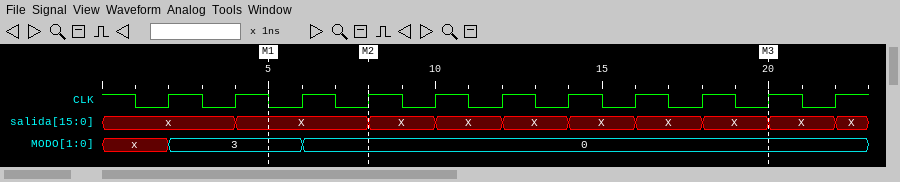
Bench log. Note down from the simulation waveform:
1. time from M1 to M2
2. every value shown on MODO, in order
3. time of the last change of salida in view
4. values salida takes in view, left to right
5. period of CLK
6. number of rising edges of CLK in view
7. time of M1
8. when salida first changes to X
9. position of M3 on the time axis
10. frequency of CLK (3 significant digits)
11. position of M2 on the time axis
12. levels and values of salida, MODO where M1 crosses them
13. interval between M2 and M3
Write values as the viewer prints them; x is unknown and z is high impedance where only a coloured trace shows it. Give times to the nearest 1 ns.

3 ns
x, 3, 0
22 ns
x, X, X, X, X, X, X, X, X, X
2 ns
11
5 ns
4 ns
20 ns
500 MHz
8 ns
salida=X, MODO=3
12 ns
